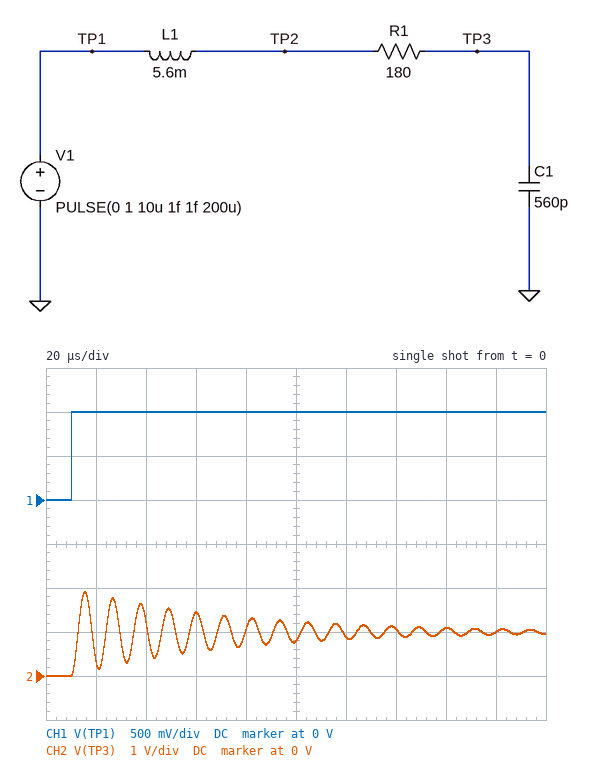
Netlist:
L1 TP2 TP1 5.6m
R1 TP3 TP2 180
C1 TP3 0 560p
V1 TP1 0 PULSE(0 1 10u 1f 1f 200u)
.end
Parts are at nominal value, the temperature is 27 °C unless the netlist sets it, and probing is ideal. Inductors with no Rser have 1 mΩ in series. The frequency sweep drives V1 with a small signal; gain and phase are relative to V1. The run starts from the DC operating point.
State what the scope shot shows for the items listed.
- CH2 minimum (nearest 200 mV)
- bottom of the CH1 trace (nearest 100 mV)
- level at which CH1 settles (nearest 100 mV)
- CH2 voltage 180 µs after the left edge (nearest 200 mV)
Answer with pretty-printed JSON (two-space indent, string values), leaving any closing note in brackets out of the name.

{
  "CH2 minimum": "0 V",
  "bottom of the CH1 trace": "0 V",
  "level at which CH1 settles": "1.0 V",
  "CH2 voltage 180 µs after the left edge": "1.0 V"
}
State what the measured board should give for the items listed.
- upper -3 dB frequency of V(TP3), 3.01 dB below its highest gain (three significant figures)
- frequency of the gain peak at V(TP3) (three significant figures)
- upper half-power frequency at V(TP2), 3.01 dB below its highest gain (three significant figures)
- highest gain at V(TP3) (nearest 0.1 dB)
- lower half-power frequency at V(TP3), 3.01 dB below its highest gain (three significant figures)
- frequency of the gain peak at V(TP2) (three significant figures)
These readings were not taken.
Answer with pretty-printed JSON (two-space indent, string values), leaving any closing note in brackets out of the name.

{
  "upper -3 dB frequency of V(TP3), 3.01 dB below its highest gain": "92.3 kHz",
  "frequency of the gain peak at V(TP3)": "89.8 kHz",
  "upper half-power frequency at V(TP2), 3.01 dB below its highest gain": "92.3 kHz",
  "highest gain at V(TP3)": "24.9 dB",
  "lower half-power frequency at V(TP3), 3.01 dB below its highest gain": "87.2 kHz",
  "frequency of the gain peak at V(TP2)": "89.8 kHz"
}
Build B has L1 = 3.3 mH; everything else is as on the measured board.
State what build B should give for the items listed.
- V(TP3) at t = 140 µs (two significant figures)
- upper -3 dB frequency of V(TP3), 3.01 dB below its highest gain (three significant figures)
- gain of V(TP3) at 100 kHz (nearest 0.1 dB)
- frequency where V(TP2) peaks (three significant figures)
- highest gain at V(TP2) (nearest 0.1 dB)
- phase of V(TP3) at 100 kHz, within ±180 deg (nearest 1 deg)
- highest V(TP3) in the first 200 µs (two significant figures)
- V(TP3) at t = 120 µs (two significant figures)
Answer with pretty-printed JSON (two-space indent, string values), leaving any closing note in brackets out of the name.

{
  "V(TP3) at t = 140 µs": "990 mV",
  "upper -3 dB frequency of V(TP3), 3.01 dB below its highest gain": "121 kHz",
  "gain of V(TP3) at 100 kHz": "11.1 dB",
  "frequency where V(TP2) peaks": "117 kHz",
  "highest gain at V(TP2)": "22.6 dB",
  "phase of V(TP3) at 100 kHz, within ±180 deg": "-13 deg",
  "highest V(TP3) in the first 200 µs": "1.9 V",
  "V(TP3) at t = 120 µs": "970 mV"
}
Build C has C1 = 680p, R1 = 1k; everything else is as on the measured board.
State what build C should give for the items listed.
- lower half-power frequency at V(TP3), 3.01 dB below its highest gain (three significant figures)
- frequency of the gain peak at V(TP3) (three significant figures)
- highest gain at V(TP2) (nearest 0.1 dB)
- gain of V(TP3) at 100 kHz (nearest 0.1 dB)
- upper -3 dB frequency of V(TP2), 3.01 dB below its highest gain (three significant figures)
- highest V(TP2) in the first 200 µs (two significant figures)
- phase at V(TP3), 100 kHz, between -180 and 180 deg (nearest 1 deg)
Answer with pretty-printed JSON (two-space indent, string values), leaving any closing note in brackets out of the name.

{
  "lower half-power frequency at V(TP3), 3.01 dB below its highest gain": "63.0 kHz",
  "frequency of the gain peak at V(TP3)": "79.0 kHz",
  "highest gain at V(TP2)": "9.8 dB",
  "gain of V(TP3) at 100 kHz": "3.6 dB",
  "upper -3 dB frequency of V(TP2), 3.01 dB below its highest gain": "92.8 kHz",
  "highest V(TP2) in the first 200 µs": "1.6 V",
  "phase at V(TP3), 100 kHz, between -180 and 180 deg": "-140 deg"
}
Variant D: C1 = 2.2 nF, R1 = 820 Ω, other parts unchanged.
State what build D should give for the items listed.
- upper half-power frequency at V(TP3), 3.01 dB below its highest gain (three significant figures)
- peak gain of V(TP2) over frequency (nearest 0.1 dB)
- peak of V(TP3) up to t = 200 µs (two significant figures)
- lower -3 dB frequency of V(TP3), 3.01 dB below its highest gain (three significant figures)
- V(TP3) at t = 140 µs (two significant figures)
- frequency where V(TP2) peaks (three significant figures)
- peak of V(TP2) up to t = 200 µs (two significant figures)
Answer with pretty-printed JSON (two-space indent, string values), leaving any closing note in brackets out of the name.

{
  "upper half-power frequency at V(TP3), 3.01 dB below its highest gain": "53.0 kHz",
  "peak gain of V(TP2) over frequency": "7.0 dB",
  "peak of V(TP3) up to t = 200 µs": "1.4 V",
  "lower -3 dB frequency of V(TP3), 3.01 dB below its highest gain": "27.6 kHz",
  "V(TP3) at t = 140 µs": "1.0 V",
  "frequency where V(TP2) peaks": "42.9 kHz",
  "peak of V(TP2) up to t = 200 µs": "1.5 V"
}
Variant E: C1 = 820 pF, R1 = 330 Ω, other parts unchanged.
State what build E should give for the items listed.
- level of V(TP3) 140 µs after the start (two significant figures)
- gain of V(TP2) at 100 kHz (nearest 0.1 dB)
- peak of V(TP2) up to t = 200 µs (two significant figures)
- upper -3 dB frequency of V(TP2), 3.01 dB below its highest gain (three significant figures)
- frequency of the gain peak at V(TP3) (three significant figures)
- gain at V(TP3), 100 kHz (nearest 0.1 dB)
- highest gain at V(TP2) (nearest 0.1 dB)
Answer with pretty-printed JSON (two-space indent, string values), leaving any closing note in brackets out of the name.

{
  "level of V(TP3) 140 µs after the start": "1.0 V",
  "gain of V(TP2) at 100 kHz": "1.7 dB",
  "peak of V(TP2) up to t = 200 µs": "1.8 V",
  "upper -3 dB frequency of V(TP2), 3.01 dB below its highest gain": "78.5 kHz",
  "frequency of the gain peak at V(TP3)": "74.0 kHz",
  "gain at V(TP3), 100 kHz": "1.6 dB",
  "highest gain at V(TP2)": "18.1 dB"
}
